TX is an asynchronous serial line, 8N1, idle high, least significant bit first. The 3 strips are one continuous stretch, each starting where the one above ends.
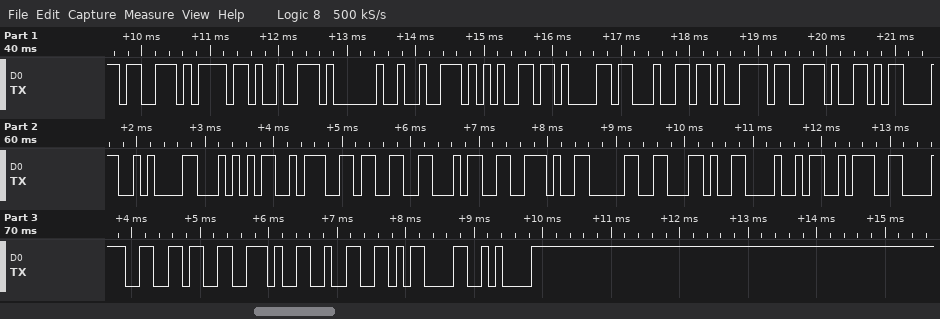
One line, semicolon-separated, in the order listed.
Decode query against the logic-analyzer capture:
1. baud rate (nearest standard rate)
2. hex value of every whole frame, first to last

9600 baud; 73 6F 72 20 72 65 61 64 79 2E 0D 0A 54 3A 33 34 2E 30 2C 48 3A 38 36 2E 32 0D 0A
